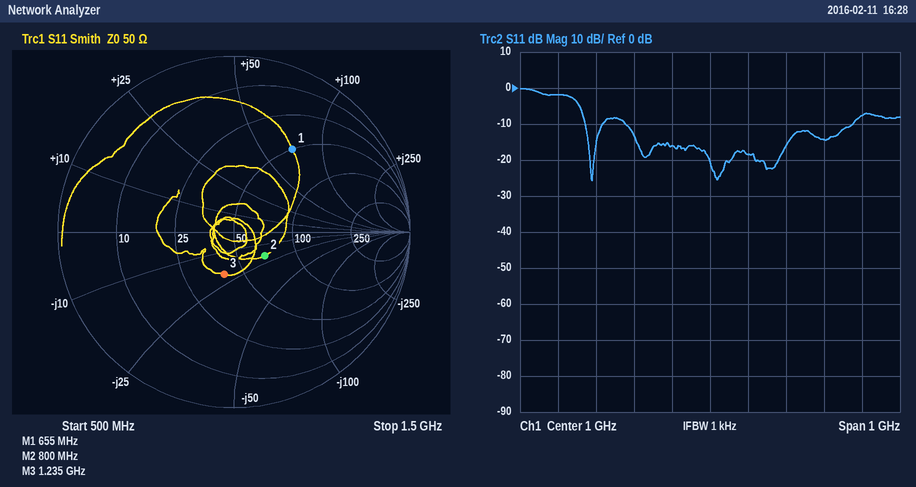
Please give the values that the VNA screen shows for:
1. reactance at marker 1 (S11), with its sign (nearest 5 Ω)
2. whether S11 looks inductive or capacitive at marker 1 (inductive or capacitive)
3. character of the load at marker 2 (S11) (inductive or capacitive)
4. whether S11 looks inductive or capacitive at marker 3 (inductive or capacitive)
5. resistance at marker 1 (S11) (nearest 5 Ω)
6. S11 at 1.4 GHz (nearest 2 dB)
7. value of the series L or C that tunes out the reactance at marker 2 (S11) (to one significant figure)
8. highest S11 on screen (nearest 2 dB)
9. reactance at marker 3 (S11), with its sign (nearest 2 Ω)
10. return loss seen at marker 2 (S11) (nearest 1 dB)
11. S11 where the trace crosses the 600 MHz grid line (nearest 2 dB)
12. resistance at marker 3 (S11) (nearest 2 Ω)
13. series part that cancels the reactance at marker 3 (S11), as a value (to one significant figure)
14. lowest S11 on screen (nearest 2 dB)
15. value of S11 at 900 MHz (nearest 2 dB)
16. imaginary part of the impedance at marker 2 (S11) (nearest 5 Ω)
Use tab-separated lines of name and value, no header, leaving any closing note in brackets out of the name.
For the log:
reactance at marker 1 (S11), with its sign	+70 Ω
whether S11 looks inductive or capacitive at marker 1	inductive
character of the load at marker 2 (S11)	capacitive
whether S11 looks inductive or capacitive at marker 3	capacitive
resistance at marker 1 (S11)	50 Ω
S11 at 1.4 GHz	-8 dB
value of the series L or C that tunes out the reactance at marker 2 (S11)	4 nH
highest S11 on screen	0 dB
reactance at marker 3 (S11), with its sign	-20 Ω
return loss seen at marker 2 (S11)	13 dB
S11 where the trace crosses the 600 MHz grid line	-2 dB
resistance at marker 3 (S11)	40 Ω
series part that cancels the reactance at marker 3 (S11), as a value	3 nH
lowest S11 on screen	-26 dB
value of S11 at 900 MHz	-16 dB
imaginary part of the impedance at marker 2 (S11)	-20 Ω
